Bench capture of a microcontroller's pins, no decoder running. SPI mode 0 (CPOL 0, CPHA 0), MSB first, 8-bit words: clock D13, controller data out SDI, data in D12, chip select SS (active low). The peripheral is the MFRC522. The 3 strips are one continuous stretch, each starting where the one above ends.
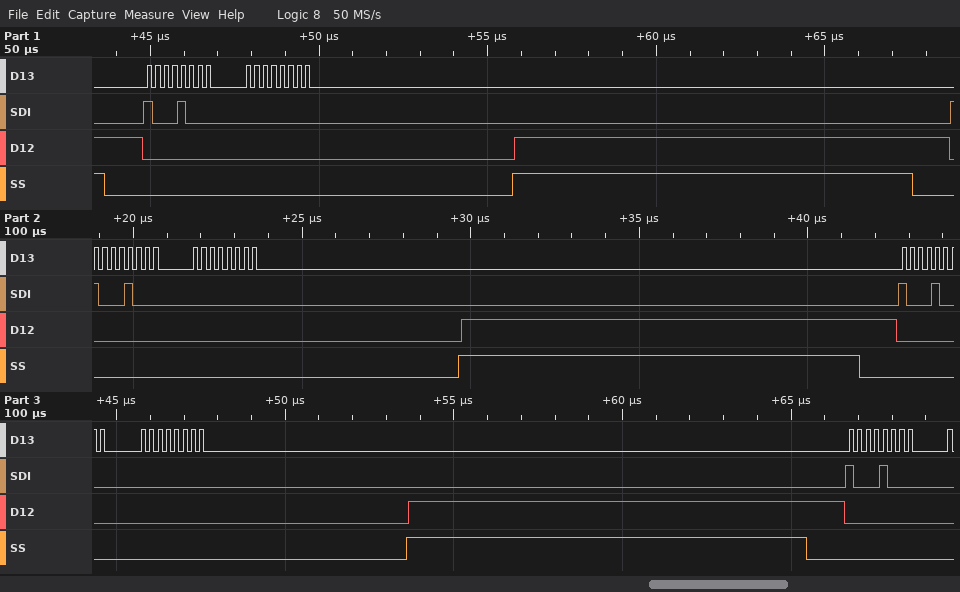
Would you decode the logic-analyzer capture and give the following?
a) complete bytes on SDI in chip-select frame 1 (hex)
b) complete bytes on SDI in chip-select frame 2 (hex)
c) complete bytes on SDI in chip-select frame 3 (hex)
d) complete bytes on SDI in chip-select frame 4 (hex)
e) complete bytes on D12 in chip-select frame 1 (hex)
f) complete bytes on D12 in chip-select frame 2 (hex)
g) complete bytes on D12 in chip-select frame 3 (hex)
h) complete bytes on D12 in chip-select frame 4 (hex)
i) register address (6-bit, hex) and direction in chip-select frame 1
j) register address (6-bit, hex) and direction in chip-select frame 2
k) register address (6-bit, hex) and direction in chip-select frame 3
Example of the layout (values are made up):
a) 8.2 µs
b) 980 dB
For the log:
a) 0x88 0x00
b) 0x88 0x00
c) 0x88 0x00
d) 0x88
e) 0x00 0x00
f) 0x00 0x00
g) 0x00 0x00
h) 0x00
i) 0x04 read
j) 0x04 read
k) 0x04 read
